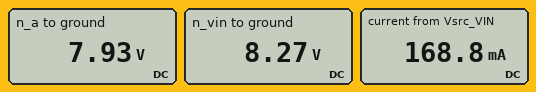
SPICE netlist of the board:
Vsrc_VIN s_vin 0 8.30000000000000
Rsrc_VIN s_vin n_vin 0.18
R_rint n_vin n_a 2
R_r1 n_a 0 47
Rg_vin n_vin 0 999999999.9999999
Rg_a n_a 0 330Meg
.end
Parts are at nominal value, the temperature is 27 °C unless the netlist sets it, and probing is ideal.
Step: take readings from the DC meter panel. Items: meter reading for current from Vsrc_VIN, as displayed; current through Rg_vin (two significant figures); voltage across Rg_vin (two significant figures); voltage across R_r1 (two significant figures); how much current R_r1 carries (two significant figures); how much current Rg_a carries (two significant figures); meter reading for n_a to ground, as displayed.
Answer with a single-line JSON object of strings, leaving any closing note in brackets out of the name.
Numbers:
{"meter reading for current from Vsrc_VIN, as displayed": "168.8 mA", "current through Rg_vin": "8.3 nA", "voltage across Rg_vin": "8.3 V", "voltage across R_r1": "7.9 V", "how much current R_r1 carries": "170 mA", "how much current Rg_a carries": "24 nA", "meter reading for n_a to ground, as displayed": "7.93 V"}
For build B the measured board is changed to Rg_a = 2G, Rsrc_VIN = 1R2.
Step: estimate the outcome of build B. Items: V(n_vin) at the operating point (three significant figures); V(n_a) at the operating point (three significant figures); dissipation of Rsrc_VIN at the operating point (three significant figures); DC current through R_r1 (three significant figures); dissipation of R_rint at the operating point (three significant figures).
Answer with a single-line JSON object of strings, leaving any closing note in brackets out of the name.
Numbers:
{"V(n_vin) at the operating point": "8.10 V", "V(n_a) at the operating point": "7.77 V", "dissipation of Rsrc_VIN at the operating point": "32.8 mW", "DC current through R_r1": "165 mA", "dissipation of R_rint at the operating point": "54.7 mW"}
